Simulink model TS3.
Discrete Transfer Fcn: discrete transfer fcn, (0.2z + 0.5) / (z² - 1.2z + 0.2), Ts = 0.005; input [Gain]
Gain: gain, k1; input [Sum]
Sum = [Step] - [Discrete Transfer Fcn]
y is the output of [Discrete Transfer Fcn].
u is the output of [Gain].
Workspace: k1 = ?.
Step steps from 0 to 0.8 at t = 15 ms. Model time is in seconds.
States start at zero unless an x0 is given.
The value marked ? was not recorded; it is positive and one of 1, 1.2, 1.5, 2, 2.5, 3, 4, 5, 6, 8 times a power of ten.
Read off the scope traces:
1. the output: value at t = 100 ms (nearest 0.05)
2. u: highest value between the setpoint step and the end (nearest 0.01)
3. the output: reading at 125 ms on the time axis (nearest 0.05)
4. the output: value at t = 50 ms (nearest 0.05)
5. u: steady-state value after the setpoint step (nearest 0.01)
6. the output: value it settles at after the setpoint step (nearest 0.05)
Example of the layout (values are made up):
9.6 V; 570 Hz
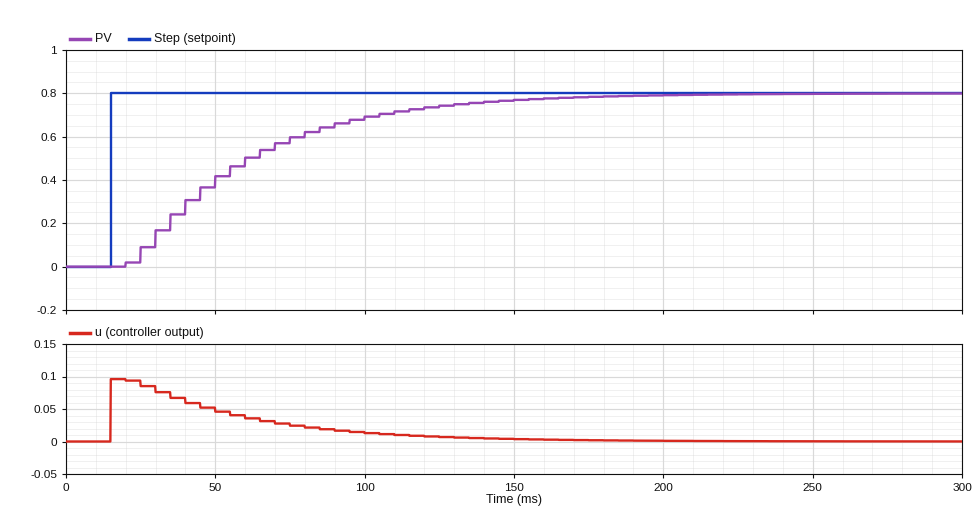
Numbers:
0.70; 0.10; 0.75; 0.40; 0.00; 0.80
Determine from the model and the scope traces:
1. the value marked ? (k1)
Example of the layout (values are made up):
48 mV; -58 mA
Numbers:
0.12
